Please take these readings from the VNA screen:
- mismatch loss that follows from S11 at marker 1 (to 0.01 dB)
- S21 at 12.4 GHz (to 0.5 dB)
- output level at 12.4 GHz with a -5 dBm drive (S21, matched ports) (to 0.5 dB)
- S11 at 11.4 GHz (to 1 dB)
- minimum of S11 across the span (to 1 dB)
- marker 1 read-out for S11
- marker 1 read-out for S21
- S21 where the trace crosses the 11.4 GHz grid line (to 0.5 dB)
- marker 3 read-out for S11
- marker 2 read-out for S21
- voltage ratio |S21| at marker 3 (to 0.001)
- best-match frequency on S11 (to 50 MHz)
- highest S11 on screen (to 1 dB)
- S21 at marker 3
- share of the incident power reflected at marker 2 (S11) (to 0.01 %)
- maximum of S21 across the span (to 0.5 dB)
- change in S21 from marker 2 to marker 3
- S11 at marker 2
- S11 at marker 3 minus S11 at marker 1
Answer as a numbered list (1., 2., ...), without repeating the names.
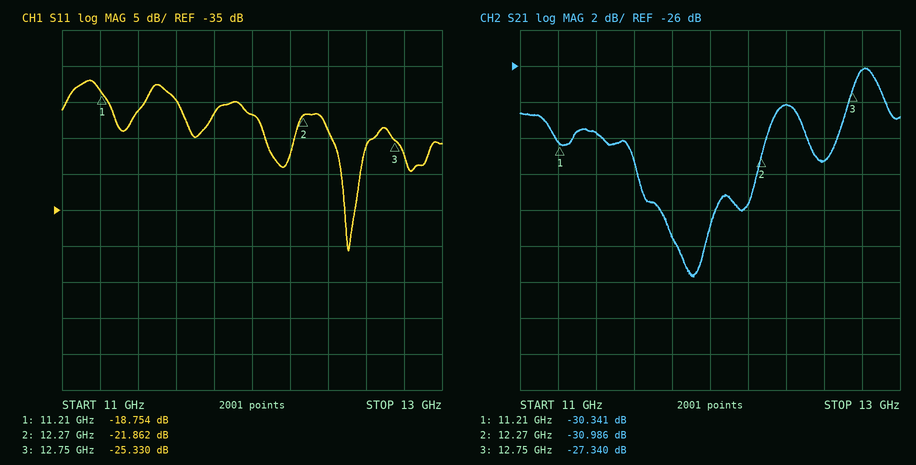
1. 0.06 dB
2. -28.0 dB
3. -33.0 dBm
4. -21 dB
5. -41 dB
6. -18.754 dB
7. -30.341 dB
8. -29.5 dB
9. -25.330 dB
10. -30.986 dB
11. 0.043
12. 12.50 GHz
13. -17 dB
14. -27.340 dB
15. 0.65 %
16. -26.0 dB
17. 3.646 dB
18. -21.862 dB
19. -6.576 dB
